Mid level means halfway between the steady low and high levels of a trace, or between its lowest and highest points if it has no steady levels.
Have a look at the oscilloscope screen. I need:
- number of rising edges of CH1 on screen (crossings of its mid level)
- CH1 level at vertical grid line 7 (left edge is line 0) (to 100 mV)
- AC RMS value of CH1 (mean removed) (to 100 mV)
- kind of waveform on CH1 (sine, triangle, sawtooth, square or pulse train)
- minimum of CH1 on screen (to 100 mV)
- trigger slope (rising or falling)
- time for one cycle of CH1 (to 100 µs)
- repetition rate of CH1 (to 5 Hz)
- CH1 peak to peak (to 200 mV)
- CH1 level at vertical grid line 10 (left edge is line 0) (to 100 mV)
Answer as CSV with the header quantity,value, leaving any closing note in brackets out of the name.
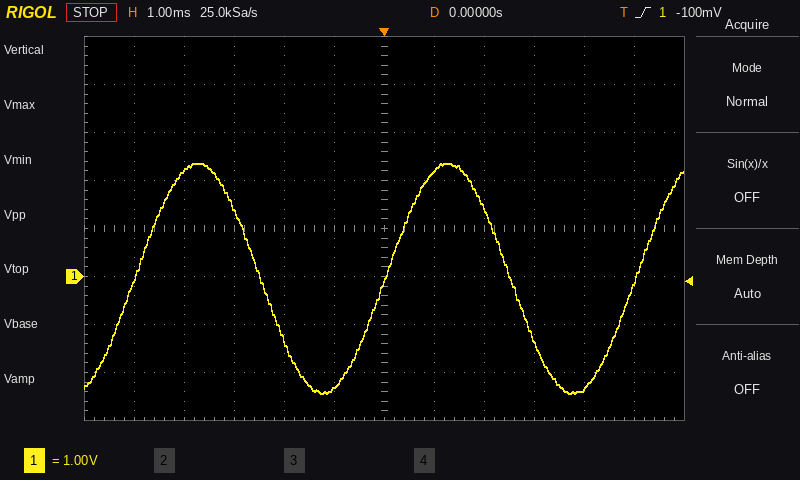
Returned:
quantity,value
number of rising edges of CH1 on screen,3
CH1 level at vertical grid line 7 (left edge is line 0),2.2 V
AC RMS value of CH1 (mean removed),1.7 V
kind of waveform on CH1,sine
minimum of CH1 on screen,-2.4 V
trigger slope,rising
time for one cycle of CH1,5.0 ms
repetition rate of CH1,200 Hz
CH1 peak to peak,4.8 V
CH1 level at vertical grid line 10 (left edge is line 0),-2.3 V
